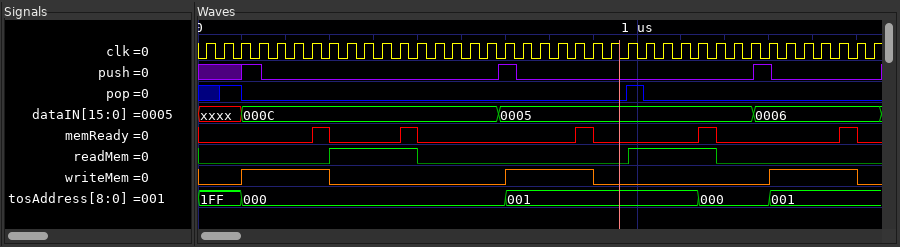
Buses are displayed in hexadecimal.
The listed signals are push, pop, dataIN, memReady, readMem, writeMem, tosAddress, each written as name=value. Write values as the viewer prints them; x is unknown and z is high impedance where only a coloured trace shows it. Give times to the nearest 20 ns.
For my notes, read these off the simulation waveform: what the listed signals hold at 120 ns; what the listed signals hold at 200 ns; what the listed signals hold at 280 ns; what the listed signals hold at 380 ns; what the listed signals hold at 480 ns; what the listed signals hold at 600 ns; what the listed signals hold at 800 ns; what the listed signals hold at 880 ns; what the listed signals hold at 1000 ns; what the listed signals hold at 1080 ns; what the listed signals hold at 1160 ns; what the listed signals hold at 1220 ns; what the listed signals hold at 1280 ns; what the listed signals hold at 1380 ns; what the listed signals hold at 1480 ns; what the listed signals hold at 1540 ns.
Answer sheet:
push=1, pop=0, dataIN=000C, memReady=0, readMem=0, writeMem=1, tosAddress=000
push=0, pop=0, dataIN=000C, memReady=0, readMem=0, writeMem=1, tosAddress=000
push=0, pop=0, dataIN=000C, memReady=1, readMem=0, writeMem=1, tosAddress=000
push=0, pop=0, dataIN=000C, memReady=0, readMem=1, writeMem=0, tosAddress=000
push=0, pop=0, dataIN=000C, memReady=1, readMem=1, writeMem=0, tosAddress=000
push=0, pop=0, dataIN=000C, memReady=0, readMem=0, writeMem=0, tosAddress=000
push=0, pop=0, dataIN=0005, memReady=0, readMem=0, writeMem=1, tosAddress=001
push=0, pop=0, dataIN=0005, memReady=1, readMem=0, writeMem=1, tosAddress=001
push=0, pop=1, dataIN=0005, memReady=0, readMem=1, writeMem=0, tosAddress=001
push=0, pop=0, dataIN=0005, memReady=0, readMem=1, writeMem=0, tosAddress=001
push=0, pop=0, dataIN=0005, memReady=1, readMem=1, writeMem=0, tosAddress=000
push=0, pop=0, dataIN=0005, memReady=0, readMem=0, writeMem=0, tosAddress=000
push=1, pop=0, dataIN=0006, memReady=0, readMem=0, writeMem=0, tosAddress=000
push=0, pop=0, dataIN=0006, memReady=0, readMem=0, writeMem=1, tosAddress=001
push=0, pop=0, dataIN=0006, memReady=1, readMem=0, writeMem=1, tosAddress=001
push=0, pop=0, dataIN=0006, memReady=0, readMem=0, writeMem=0, tosAddress=001
